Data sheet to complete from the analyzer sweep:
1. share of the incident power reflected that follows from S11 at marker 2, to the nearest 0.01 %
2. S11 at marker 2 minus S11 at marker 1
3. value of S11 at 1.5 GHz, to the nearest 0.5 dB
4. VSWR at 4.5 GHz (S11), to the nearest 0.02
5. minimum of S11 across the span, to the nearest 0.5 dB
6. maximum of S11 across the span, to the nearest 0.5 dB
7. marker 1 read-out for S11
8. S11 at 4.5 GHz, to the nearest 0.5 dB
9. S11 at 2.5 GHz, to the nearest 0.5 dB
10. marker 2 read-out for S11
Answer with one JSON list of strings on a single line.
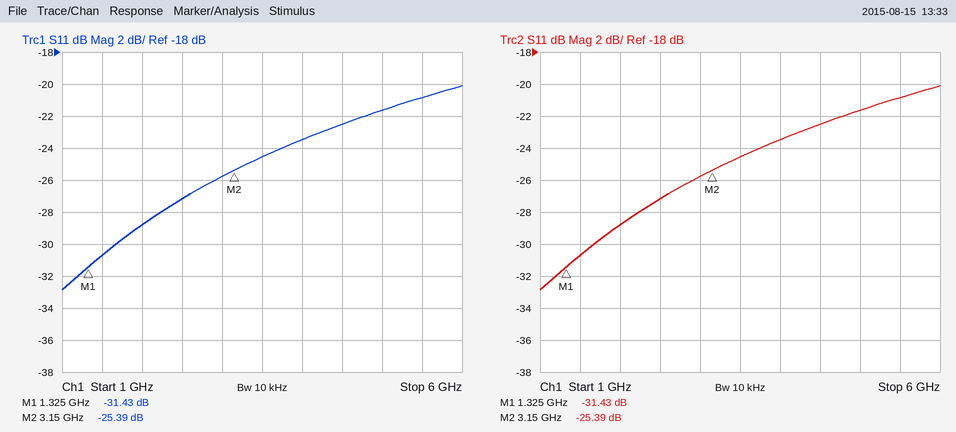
["0.29 %", "6.04 dB", "-30.5 dB", "1.16", "-33.0 dB", "-20.0 dB", "-31.43 dB", "-22.5 dB", "-27.0 dB", "-25.39 dB"]
